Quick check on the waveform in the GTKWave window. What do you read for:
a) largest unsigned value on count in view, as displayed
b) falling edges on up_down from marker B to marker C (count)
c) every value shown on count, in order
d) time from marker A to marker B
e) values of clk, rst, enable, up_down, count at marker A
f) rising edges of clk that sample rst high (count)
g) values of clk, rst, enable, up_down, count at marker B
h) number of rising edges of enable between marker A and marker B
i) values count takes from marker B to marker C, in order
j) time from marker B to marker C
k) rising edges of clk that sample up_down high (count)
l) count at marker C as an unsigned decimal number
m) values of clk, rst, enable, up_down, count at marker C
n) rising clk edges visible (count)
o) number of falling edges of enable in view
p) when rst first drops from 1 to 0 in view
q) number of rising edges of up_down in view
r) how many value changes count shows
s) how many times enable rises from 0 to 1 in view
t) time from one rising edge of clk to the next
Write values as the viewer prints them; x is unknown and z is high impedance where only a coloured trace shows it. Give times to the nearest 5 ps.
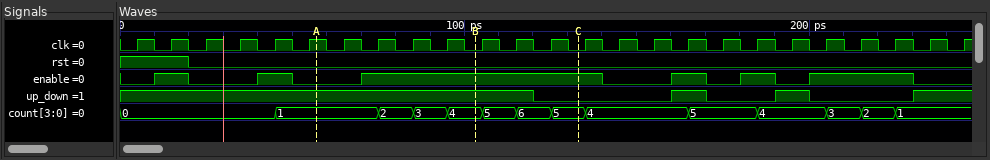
6
1
0, 1, 2, 3, 4, 5, 6, 5, 4, 5, 4, 3, 2, 1
45 ps
clk=1, rst=0, enable=0, up_down=1, count=1
2
clk=0, rst=0, enable=1, up_down=1, count=4
1
4, 5, 6, 5
30 ps
16
5
clk=0, rst=0, enable=1, up_down=0, count=5
25
6
20 ps
3
13
6
10 ps
